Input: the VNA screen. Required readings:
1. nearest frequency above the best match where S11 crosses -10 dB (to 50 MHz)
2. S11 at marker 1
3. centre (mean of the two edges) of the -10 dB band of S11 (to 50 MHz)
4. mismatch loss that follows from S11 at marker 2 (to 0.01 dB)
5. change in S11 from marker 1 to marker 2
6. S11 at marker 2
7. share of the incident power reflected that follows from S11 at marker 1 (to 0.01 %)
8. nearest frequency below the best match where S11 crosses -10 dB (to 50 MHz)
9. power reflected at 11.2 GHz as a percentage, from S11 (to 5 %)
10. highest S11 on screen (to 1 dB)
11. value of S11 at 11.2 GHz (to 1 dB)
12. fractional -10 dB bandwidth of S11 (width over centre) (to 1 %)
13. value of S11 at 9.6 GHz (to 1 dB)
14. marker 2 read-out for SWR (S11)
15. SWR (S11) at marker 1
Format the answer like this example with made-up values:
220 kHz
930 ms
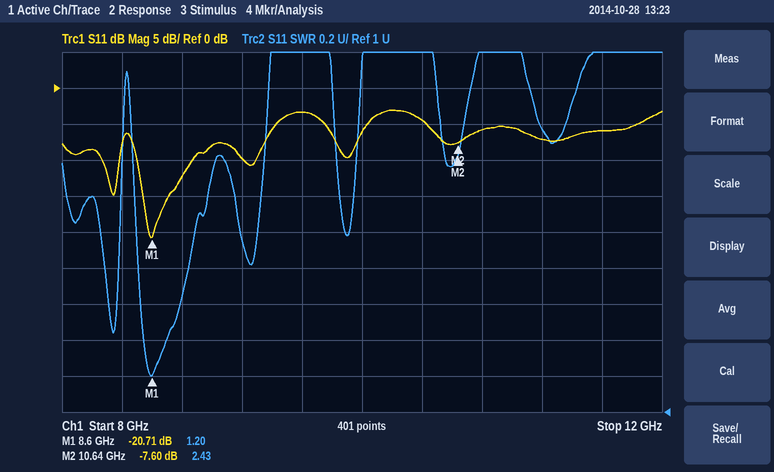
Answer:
8.85 GHz
-20.71 dB
8.70 GHz
0.83 dB
13.11 dB
-7.60 dB
0.85 %
8.50 GHz
20 %
-3 dB
-7 dB
4 %
-3 dB
2.43
1.20
